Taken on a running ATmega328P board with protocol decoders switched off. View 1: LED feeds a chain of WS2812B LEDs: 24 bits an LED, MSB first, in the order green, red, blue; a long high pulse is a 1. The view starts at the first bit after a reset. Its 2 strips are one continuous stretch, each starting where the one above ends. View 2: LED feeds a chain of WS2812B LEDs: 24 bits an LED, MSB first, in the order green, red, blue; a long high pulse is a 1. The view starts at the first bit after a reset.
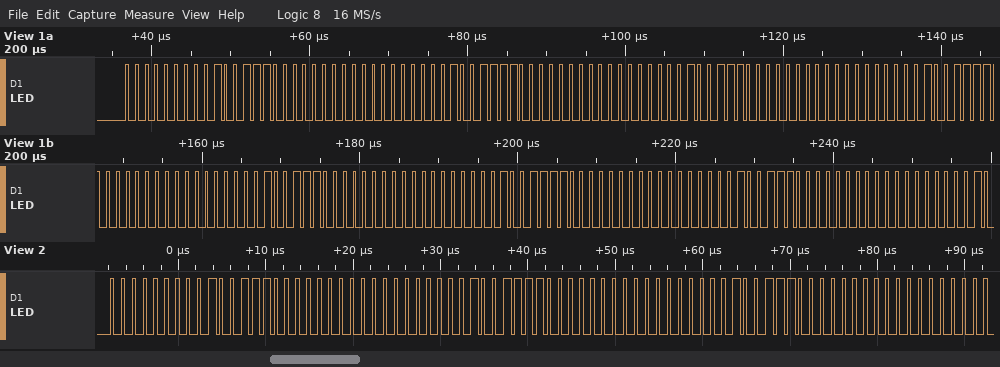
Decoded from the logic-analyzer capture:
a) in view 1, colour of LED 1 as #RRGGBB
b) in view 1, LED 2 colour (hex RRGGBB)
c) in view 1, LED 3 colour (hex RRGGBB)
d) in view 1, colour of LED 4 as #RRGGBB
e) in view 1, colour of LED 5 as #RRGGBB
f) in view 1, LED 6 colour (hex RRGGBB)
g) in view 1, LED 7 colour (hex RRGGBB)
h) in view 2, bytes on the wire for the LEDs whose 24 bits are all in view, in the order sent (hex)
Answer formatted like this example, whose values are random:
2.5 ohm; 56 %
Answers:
#4E0000; #4F0000; #4E0000; #4F0000; #4E0000; #4F0000; #4E0000; 00 4E 00 00 4F 00 00 4E 00
